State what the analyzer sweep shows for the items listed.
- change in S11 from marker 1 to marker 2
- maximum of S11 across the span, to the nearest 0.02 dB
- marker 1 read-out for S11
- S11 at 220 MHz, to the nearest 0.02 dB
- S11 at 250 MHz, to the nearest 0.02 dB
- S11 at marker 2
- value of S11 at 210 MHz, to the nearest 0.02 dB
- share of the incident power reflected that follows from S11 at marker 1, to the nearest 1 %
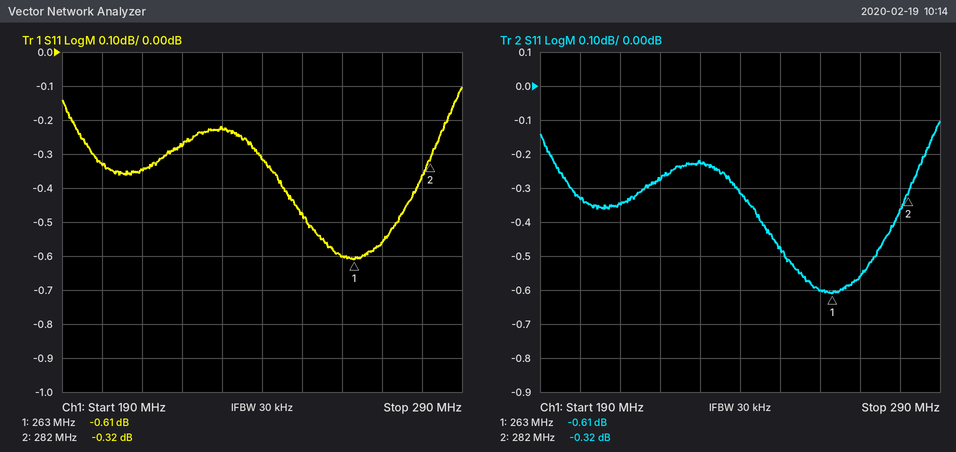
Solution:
0.29 dB
-0.10 dB
-0.61 dB
-0.28 dB
-0.48 dB
-0.32 dB
-0.34 dB
87 %
